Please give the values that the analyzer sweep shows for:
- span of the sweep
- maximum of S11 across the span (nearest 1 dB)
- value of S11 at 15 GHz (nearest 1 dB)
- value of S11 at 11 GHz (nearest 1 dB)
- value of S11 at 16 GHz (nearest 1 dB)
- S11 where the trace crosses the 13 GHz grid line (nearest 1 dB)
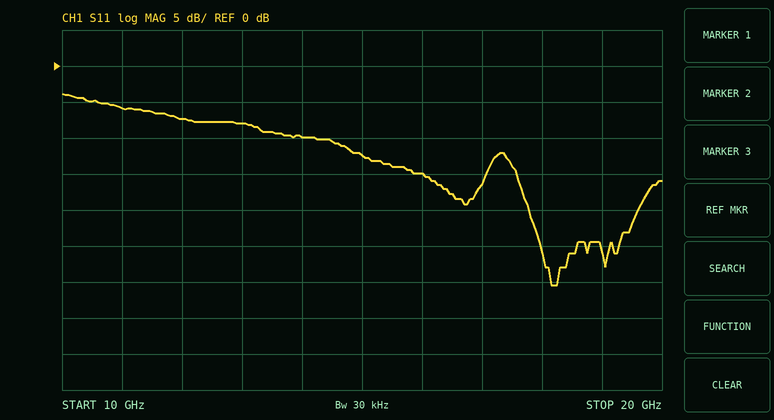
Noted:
10 GHz
-4 dB
-12 dB
-6 dB
-15 dB
-8 dB
